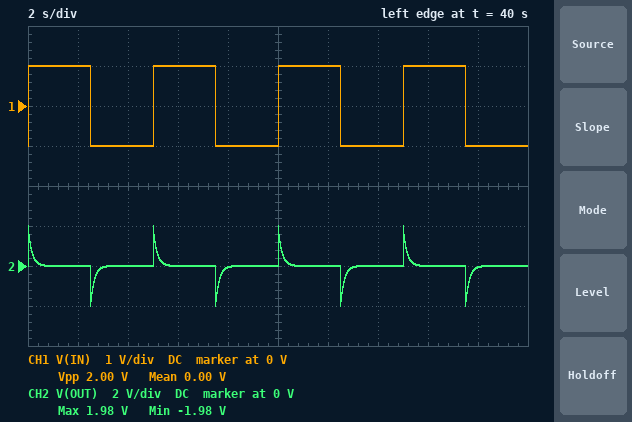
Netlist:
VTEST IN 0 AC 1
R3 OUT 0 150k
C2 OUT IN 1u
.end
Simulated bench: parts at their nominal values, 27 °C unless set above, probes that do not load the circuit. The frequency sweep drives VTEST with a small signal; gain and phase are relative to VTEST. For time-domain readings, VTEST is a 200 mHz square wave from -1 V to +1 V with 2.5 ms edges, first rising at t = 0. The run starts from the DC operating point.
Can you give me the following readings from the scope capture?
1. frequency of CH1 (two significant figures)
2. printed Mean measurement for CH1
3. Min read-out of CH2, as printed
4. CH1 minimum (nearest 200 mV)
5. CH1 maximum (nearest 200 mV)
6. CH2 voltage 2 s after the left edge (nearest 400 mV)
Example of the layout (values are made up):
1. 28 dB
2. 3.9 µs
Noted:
1. 200 mHz
2. 0.00 V
3. -1.98 V
4. -1.0 V
5. 1.0 V
6. 0 V
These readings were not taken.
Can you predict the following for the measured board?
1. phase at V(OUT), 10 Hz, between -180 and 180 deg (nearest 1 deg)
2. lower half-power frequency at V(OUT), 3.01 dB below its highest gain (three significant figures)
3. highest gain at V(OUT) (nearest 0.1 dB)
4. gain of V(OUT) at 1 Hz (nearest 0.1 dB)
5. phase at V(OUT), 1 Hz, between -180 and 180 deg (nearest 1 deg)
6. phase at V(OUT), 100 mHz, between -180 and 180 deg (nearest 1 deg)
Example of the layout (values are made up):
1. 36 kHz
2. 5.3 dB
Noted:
1. 6 deg
2. 1.06 Hz
3. 0 dB
4. -3.3 dB
5. 47 deg
6. 85 deg
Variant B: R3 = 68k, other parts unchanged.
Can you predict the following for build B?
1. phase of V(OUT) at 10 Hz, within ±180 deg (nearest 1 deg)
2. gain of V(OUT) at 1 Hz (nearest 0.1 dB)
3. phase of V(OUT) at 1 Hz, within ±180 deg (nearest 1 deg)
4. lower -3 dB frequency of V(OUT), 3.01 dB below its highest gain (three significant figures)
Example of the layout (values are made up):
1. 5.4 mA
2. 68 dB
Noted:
1. 13 deg
2. -8.1 dB
3. 67 deg
4. 2.34 Hz
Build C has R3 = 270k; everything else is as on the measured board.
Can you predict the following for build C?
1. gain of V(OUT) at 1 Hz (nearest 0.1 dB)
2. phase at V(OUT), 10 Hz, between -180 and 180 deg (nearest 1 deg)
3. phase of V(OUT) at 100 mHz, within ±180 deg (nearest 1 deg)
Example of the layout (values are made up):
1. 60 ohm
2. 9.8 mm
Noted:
1. -1.3 dB
2. 3 deg
3. 80 deg
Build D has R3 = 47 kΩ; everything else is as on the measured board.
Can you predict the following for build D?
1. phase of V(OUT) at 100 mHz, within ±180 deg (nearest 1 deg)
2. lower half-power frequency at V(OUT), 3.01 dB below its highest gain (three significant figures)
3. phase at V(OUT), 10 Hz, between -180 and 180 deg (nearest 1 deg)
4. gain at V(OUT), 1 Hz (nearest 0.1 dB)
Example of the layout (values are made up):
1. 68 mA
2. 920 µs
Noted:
1. 88 deg
2. 3.39 Hz
3. 19 deg
4. -11.0 dB
